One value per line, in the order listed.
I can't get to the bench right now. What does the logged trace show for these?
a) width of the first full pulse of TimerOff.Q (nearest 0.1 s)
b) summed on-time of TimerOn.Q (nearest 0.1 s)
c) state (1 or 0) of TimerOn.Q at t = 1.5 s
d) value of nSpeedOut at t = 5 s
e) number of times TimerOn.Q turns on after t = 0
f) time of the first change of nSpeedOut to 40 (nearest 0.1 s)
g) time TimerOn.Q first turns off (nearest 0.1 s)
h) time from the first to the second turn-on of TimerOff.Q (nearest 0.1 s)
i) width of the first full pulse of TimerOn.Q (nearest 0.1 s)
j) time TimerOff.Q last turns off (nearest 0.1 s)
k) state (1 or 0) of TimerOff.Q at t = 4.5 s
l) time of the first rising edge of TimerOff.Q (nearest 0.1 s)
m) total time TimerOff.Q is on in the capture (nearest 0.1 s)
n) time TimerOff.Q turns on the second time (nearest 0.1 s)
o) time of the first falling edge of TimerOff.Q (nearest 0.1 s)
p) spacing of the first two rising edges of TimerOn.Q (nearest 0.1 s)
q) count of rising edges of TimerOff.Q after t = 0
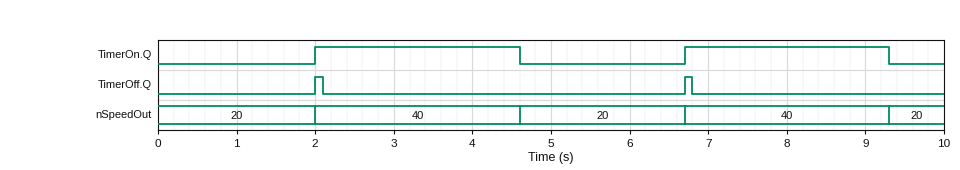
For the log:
0.1 s
5.2 s
0
20
2
2.0 s
4.6 s
4.7 s
2.6 s
6.8 s
0
2.0 s
0.2 s
6.7 s
2.1 s
4.7 s
2
